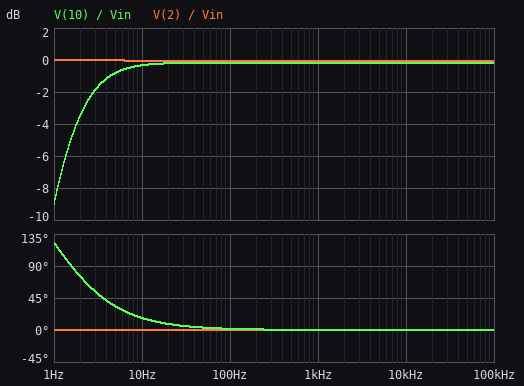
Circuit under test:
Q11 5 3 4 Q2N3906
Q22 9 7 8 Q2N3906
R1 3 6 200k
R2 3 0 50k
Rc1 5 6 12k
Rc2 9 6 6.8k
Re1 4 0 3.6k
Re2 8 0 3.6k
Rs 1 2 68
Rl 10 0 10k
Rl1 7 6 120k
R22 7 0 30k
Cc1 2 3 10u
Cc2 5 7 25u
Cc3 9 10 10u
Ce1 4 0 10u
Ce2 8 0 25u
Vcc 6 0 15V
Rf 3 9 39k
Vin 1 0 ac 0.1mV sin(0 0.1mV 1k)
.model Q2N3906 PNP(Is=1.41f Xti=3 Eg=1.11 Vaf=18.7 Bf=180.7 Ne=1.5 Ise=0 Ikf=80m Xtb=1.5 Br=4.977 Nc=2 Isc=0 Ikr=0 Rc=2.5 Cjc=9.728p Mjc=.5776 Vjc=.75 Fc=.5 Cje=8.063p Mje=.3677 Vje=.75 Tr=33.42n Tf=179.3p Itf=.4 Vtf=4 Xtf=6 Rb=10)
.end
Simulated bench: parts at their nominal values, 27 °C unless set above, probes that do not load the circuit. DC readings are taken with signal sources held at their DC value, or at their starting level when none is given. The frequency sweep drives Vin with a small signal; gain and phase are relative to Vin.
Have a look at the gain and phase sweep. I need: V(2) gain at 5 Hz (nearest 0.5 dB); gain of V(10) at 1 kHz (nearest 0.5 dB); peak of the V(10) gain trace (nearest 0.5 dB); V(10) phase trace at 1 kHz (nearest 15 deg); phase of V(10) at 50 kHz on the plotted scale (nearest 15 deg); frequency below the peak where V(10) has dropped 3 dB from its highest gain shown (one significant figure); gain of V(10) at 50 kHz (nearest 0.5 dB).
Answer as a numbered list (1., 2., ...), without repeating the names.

1. 0 dB
2. 0 dB
3. 0 dB
4. 0 deg
5. 0 deg
6. 2 Hz
7. 0 dB
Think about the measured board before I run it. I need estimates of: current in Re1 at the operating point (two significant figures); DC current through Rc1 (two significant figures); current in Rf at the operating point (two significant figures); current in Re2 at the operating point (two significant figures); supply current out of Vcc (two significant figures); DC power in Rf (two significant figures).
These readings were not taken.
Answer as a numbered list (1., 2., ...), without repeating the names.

1. 470 µA
2. 570 µA
3. 13 µA
4. 850 µA
5. 1.7 mA
6. 6.3 µW
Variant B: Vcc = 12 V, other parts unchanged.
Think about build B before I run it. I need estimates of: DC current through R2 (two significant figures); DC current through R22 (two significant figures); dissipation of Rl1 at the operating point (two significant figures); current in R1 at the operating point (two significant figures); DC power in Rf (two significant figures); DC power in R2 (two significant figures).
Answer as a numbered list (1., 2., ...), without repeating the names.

1. 120 µA
2. 190 µA
3. 330 µW
4. 30 µA
5. 5.8 µW
6. 710 µW
